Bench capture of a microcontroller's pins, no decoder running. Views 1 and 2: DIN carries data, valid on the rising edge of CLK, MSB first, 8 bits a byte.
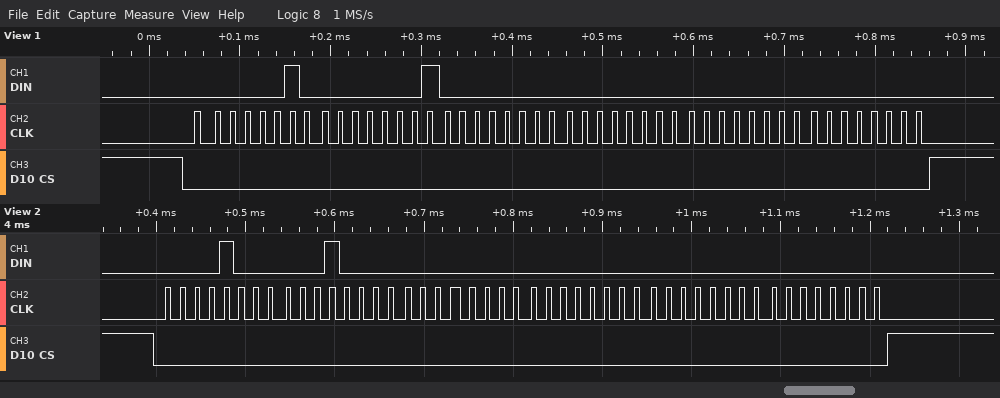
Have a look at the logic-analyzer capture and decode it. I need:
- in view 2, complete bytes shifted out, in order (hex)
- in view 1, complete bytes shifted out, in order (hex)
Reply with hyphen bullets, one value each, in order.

- 0x08 0x10 0x00 0x00 0x00 0x00
- 0x02 0x01 0x00 0x00 0x00 0x00
